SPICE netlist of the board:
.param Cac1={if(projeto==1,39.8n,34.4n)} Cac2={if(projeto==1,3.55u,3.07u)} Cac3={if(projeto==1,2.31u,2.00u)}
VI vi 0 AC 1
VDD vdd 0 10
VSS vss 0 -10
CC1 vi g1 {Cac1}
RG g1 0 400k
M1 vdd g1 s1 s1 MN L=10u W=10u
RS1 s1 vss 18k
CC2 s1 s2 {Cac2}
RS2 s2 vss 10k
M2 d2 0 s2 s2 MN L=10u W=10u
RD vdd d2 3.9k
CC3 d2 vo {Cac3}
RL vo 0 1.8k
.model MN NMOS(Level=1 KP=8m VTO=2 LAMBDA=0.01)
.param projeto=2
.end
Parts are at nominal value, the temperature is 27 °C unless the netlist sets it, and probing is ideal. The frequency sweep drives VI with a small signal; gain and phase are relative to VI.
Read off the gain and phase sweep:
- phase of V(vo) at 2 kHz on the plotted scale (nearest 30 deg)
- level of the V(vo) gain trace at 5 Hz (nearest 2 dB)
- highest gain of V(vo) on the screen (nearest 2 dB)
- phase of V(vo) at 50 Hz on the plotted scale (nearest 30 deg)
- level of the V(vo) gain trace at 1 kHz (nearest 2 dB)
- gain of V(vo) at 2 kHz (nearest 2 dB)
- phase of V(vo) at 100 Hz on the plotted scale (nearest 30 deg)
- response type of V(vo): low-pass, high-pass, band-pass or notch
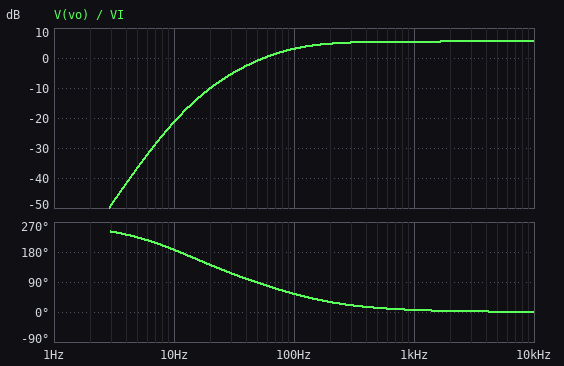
0 deg
-36 dB
6 dB
90 deg
6 dB
6 dB
60 deg
high-pass
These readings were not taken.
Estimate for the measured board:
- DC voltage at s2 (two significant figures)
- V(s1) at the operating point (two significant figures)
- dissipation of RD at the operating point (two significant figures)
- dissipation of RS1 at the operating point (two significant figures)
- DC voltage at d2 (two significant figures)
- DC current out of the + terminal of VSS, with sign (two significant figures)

-2.4 V
-2.3 V
2.2 mW
3.3 mW
7.0 V
-1.2 mA
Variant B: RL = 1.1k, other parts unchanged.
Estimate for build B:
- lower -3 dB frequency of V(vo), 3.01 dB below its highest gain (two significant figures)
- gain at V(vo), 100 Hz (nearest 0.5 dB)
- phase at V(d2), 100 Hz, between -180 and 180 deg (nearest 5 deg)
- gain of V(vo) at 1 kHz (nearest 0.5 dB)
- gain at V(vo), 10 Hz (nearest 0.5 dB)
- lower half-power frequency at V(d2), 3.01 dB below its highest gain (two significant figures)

88 Hz
0 dB
20 deg
2.5 dB
-25.5 dB
28 Hz
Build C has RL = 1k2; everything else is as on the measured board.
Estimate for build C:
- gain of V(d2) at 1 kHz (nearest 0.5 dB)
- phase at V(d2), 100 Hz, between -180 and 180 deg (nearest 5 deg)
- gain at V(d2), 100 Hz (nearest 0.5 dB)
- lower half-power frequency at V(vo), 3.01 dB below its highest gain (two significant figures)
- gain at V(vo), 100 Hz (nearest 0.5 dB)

3.0 dB
20 deg
2.0 dB
88 Hz
0.5 dB
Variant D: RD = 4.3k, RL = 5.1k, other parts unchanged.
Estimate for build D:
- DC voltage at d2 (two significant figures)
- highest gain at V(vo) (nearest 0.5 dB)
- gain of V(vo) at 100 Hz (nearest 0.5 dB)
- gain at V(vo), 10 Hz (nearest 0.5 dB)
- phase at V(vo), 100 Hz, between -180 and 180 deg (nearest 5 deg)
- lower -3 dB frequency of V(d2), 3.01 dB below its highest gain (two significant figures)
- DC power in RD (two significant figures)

6.7 V
11.0 dB
8.5 dB
-13.5 dB
50 deg
83 Hz
2.5 mW
